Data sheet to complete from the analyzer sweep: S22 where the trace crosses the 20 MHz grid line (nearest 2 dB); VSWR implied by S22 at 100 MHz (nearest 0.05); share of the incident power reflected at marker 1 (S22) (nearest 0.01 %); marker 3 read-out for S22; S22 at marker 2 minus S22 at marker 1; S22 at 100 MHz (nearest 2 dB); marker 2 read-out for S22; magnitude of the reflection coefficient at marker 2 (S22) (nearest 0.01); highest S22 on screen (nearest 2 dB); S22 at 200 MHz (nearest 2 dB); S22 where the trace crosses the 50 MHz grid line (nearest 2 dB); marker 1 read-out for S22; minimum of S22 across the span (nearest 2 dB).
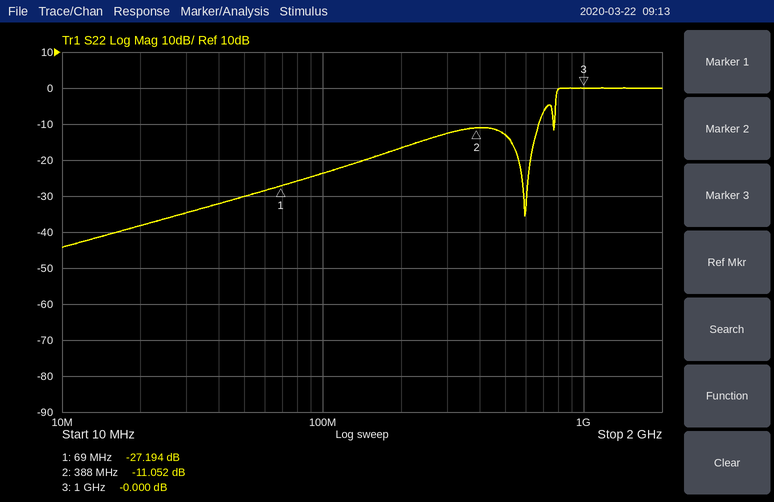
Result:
-38 dB
1.15
0.19 %
-0.000 dB
16.142 dB
-24 dB
-11.052 dB
0.28
0 dB
-16 dB
-30 dB
-27.194 dB
-44 dB
